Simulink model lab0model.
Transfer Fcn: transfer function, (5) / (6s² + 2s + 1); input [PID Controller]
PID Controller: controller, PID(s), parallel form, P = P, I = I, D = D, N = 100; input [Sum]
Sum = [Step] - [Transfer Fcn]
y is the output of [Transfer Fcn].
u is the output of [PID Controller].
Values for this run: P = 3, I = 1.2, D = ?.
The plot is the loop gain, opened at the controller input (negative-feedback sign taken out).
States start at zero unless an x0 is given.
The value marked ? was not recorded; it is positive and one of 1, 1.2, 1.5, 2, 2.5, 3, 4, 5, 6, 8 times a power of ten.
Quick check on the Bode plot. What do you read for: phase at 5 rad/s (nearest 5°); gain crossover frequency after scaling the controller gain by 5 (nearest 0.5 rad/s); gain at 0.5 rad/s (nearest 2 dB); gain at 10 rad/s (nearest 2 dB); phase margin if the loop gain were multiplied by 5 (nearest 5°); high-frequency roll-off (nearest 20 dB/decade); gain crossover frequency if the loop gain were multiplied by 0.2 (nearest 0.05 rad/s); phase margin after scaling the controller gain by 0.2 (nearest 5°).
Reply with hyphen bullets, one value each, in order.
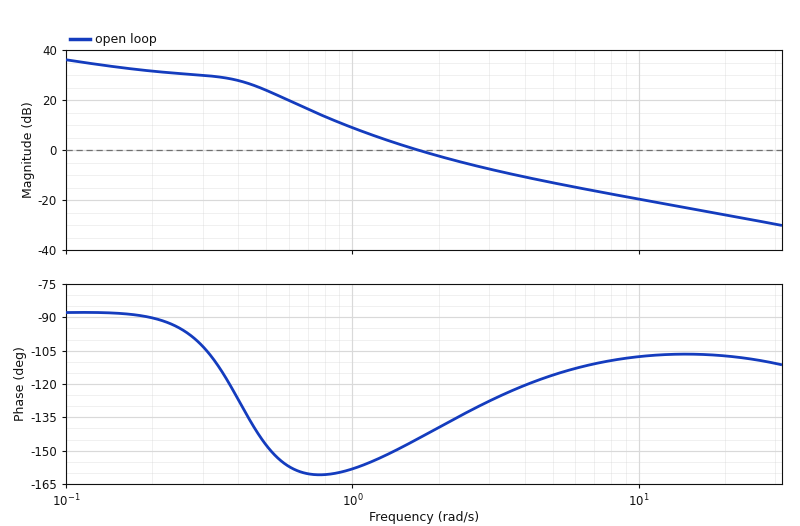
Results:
- -115°
- 5.5 rad/s
- 24 dB
- -20 dB
- 65°
- -20 dB/decade
- 0.80 rad/s
- 20°
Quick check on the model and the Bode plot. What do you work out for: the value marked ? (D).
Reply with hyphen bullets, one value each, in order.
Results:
- 1.2
